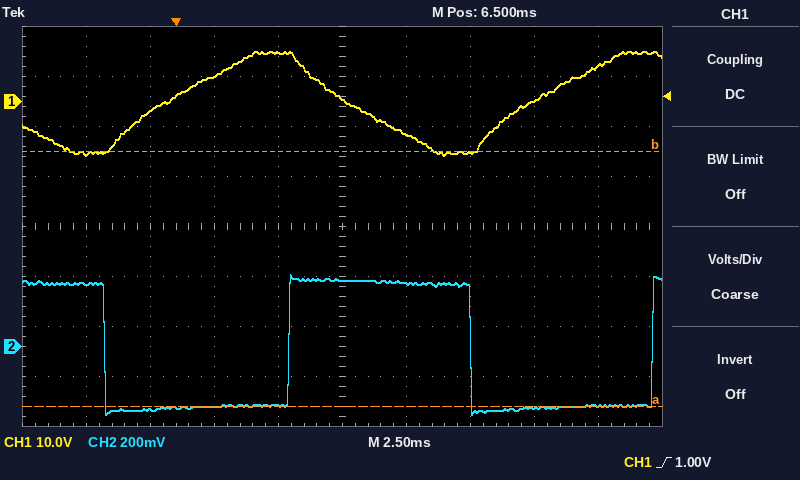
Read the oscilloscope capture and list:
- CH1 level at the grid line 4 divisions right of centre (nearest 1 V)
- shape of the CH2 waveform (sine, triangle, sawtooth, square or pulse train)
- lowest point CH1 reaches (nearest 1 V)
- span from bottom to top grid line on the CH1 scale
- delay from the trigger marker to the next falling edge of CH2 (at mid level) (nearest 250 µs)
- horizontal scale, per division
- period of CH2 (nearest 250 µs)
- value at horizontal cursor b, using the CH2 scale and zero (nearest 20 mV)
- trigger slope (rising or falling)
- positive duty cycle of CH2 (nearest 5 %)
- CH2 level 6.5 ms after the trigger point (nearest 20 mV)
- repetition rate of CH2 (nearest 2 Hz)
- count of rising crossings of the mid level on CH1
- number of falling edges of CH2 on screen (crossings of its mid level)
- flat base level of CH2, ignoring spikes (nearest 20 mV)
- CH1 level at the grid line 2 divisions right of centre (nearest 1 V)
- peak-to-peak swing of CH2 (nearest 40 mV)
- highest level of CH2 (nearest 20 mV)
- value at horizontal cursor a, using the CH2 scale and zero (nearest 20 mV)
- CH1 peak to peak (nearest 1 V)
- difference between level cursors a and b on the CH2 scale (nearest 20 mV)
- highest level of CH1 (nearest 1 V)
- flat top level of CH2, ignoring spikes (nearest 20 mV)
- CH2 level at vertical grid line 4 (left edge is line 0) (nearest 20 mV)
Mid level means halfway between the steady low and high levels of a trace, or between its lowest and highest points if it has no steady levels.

7 V
square
-11 V
80 V
11.50 ms
2.5 ms
14.25 ms
780 mV
rising
50 %
260 mV
70 Hz
2
2
-240 mV
-10 V
560 mV
280 mV
-240 mV
21 V
1.02 V
10 V
260 mV
-240 mV
